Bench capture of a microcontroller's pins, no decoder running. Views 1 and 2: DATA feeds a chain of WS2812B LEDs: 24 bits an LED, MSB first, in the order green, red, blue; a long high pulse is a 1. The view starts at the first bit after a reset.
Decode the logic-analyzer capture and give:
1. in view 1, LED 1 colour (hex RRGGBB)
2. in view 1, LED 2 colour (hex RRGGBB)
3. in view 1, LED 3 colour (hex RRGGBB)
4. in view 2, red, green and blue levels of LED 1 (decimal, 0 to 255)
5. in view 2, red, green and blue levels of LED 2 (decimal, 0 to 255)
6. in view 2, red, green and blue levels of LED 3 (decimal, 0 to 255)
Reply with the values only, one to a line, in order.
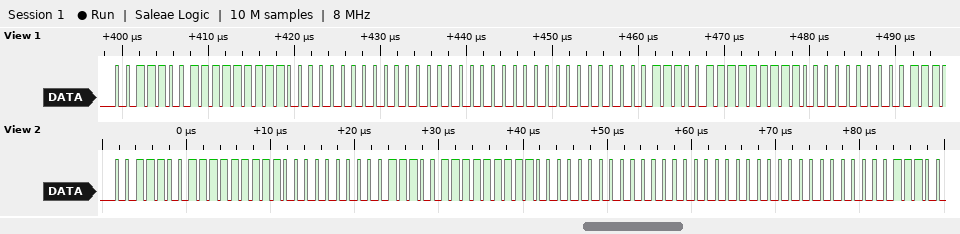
#FF3900
#000000
#FF3900
255, 57, 0
255, 57, 0
0, 0, 0
